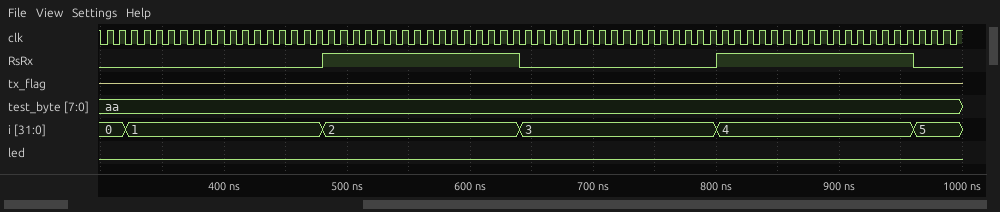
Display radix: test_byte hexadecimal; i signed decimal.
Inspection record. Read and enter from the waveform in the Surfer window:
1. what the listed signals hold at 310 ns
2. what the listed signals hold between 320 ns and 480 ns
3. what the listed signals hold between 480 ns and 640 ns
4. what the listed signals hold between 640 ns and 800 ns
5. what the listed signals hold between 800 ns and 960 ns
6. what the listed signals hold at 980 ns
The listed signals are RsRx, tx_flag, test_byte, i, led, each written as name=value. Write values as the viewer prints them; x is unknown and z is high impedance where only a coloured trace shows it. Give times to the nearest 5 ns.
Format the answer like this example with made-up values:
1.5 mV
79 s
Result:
RsRx=0, tx_flag=z, test_byte=aa, i=0, led=0
RsRx=0, tx_flag=z, test_byte=aa, i=1, led=0
RsRx=1, tx_flag=z, test_byte=aa, i=2, led=0
RsRx=0, tx_flag=z, test_byte=aa, i=3, led=0
RsRx=1, tx_flag=z, test_byte=aa, i=4, led=0
RsRx=0, tx_flag=z, test_byte=aa, i=5, led=0
